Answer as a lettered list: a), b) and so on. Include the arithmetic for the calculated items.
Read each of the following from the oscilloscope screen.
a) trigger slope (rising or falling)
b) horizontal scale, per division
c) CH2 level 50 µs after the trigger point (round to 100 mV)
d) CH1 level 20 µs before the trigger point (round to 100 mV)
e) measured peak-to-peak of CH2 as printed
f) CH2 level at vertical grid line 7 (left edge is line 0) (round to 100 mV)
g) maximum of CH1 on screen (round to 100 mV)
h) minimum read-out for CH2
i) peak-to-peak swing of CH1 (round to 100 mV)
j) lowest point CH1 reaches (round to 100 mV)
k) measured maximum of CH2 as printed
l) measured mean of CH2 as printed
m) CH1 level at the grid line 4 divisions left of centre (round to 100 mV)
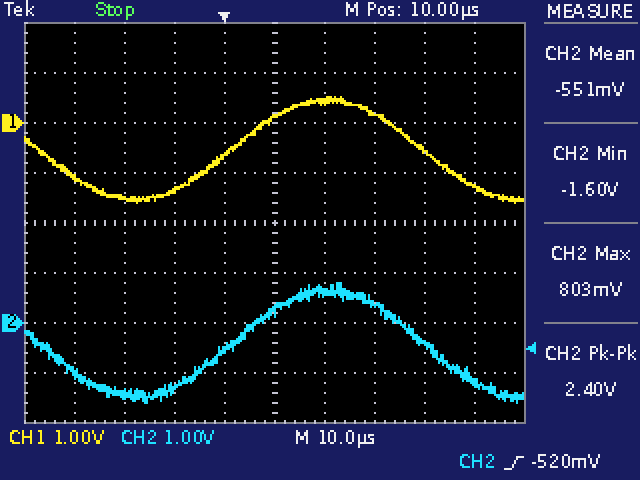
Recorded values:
a) rising
b) 10 µs
c) -1.2 V
d) -1.5 V
e) 2.40 V
f) 400 mV
g) 500 mV
h) -1.60 V
i) 500 mV − (-1.6 V) = 2.1 V
j) -1.6 V
k) 803 mV
l) -551 mV
m) -1.1 V
